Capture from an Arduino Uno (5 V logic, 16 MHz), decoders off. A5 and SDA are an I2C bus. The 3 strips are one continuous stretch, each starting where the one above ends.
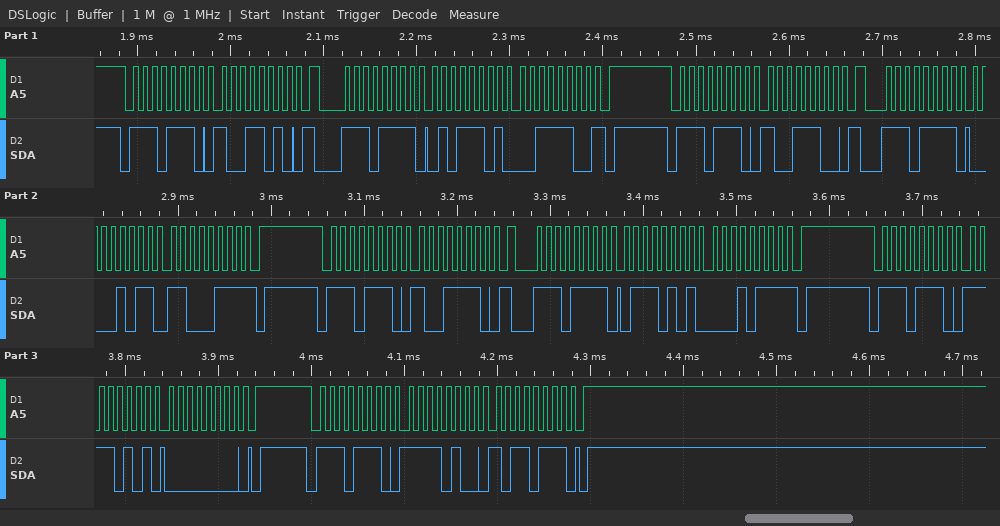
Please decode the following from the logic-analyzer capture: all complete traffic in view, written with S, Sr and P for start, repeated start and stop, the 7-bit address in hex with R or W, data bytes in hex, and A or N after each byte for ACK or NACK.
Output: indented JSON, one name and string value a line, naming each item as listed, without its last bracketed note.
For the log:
{
  "all complete traffic in view, written with S, Sr and P for start, repeated start and stop, the 7-bit address in hex with R or W, data bytes in hex, and A or N after each byte for ACK or NACK": "S 77W A 9A A Sr 77R A 5D A 3C N P S 77W A 9C A Sr 77R A 0B A C7 N P S 77W A 9E A Sr 77R A 75 A 17 N P S 77W A F5 A 00 A P S 77W A F4 A B7 A P"
}
